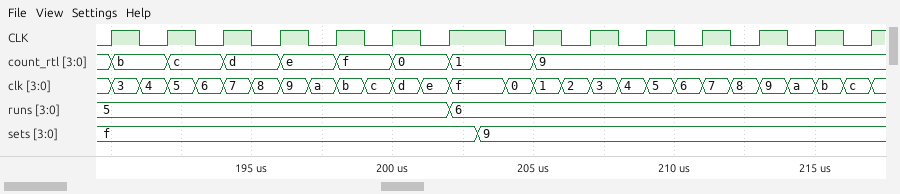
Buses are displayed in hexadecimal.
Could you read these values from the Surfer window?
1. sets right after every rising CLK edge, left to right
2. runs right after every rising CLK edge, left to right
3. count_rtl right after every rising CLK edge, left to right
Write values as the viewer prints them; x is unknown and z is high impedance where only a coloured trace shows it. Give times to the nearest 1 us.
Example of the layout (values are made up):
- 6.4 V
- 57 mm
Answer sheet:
- f, f, f, f, f, f, f, 9, 9, 9, 9, 9, 9, 9
- 5, 5, 5, 5, 5, 5, 6, 6, 6, 6, 6, 6, 6, 6
- b, c, d, e, f, 0, 1, 9, 9, 9, 9, 9, 9, 9
